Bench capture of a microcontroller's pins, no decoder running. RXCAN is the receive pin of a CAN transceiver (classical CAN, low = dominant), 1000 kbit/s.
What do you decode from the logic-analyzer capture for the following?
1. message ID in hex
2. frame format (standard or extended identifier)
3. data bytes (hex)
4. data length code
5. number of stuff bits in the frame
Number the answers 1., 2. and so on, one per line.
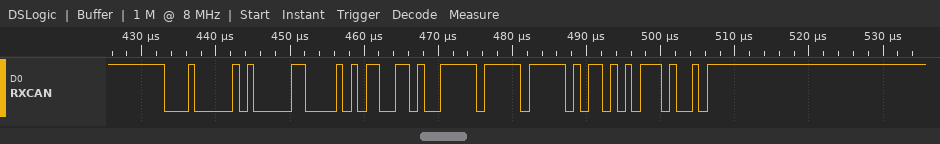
1. 0x102
2. standard
3. 2B 34 FF FF
4. 4
5. 5
